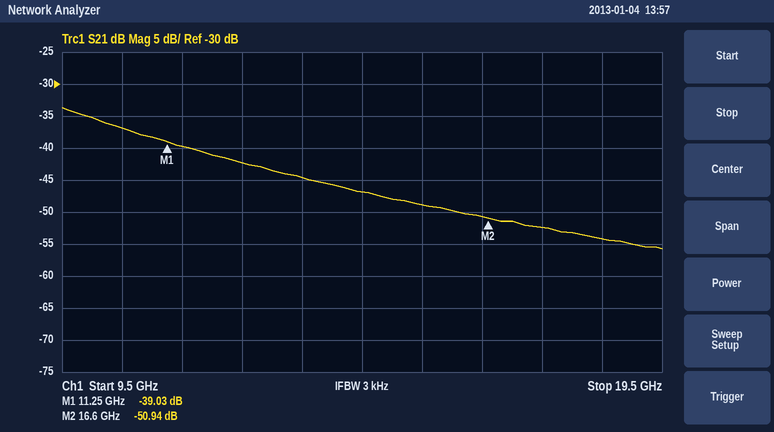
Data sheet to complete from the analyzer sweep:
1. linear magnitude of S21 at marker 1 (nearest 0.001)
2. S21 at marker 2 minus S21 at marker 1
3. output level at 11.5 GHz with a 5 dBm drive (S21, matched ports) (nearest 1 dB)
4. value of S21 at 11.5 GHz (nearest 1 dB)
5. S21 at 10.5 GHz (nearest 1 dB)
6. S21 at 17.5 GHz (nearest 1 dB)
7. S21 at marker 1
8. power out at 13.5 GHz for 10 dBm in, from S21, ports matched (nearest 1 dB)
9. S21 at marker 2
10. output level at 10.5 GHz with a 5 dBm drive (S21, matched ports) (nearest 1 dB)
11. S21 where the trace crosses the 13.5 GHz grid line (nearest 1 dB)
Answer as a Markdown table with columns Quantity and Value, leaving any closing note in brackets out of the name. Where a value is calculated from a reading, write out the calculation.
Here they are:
| Quantity | Value |
|---|---|
| linear magnitude of S21 at marker 1 | 10^(-39.03/20) ≈ 0.011 |
| S21 at marker 2 minus S21 at marker 1 | -50.94 − (-39.03) = -11.91 dB |
| output level at 11.5 GHz with a 5 dBm drive (S21, matched ports) | 5 dBm + (-40 dB) = -35 dBm |
| value of S21 at 11.5 GHz | -40 dB |
| S21 at 10.5 GHz | -37 dB |
| S21 at 17.5 GHz | -52 dB |
| S21 at marker 1 | -39.03 dB |
| power out at 13.5 GHz for 10 dBm in, from S21, ports matched | 10 dBm + (-45 dB) = -35 dBm |
| S21 at marker 2 | -50.94 dB |
| output level at 10.5 GHz with a 5 dBm drive (S21, matched ports) | 5 dBm + (-37 dB) = -32 dBm |
| S21 where the trace crosses the 13.5 GHz grid line | -45 dB |
